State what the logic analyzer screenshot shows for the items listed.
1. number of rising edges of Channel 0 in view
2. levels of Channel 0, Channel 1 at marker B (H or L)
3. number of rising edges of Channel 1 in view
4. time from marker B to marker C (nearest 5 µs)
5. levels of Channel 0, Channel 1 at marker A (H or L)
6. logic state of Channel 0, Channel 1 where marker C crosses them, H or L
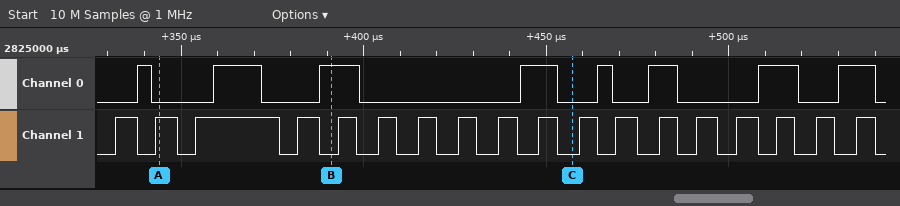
8
Channel 0=H, Channel 1=L
18
65 µs
Channel 0=L, Channel 1=H
Channel 0=L, Channel 1=L
